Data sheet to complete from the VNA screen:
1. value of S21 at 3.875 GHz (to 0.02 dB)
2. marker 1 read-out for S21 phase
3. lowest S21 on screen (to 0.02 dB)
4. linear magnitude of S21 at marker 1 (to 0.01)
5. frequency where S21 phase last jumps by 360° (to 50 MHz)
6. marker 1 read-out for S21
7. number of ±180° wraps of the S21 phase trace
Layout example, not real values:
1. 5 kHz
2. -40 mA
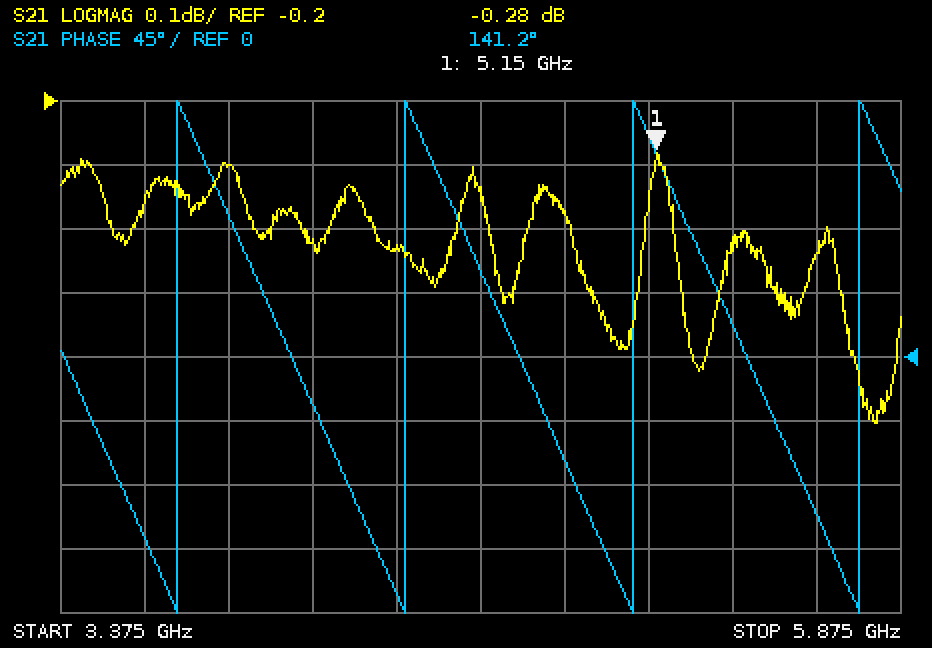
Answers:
1. -0.30 dB
2. 141.2°
3. -0.70 dB
4. 0.97
5. 5.75 GHz
6. -0.28 dB
7. 4
